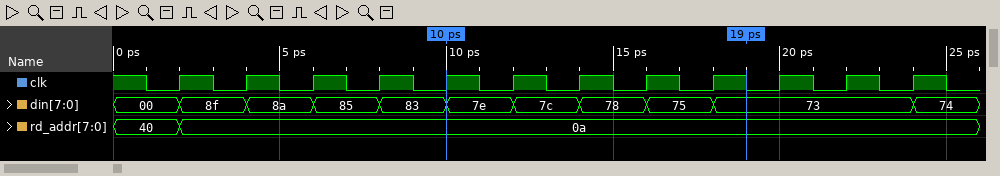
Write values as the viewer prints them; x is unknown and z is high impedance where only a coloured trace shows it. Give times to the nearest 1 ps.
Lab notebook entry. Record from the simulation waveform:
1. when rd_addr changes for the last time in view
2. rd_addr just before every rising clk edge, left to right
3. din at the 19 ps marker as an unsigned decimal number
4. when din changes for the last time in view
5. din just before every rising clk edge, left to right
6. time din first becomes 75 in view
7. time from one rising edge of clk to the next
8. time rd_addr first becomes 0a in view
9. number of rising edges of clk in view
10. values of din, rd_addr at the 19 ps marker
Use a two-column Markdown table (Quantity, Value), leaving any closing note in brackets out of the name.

| Quantity | Value |
|---|---|
| when rd_addr changes for the last time in view | 2 ps |
| rd_addr just before every rising clk edge, left to right | 40, 0a, 0a, 0a, 0a, 0a, 0a, 0a, 0a, 0a, 0a, 0a |
| din at the 19 ps marker as an unsigned decimal number | 115 |
| when din changes for the last time in view | 24 ps |
| din just before every rising clk edge, left to right | 00, 8f, 8a, 85, 83, 7e, 7c, 78, 75, 73, 73, 73 |
| time din first becomes 75 in view | 16 ps |
| time from one rising edge of clk to the next | 2 ps |
| time rd_addr first becomes 0a in view | 2 ps |
| number of rising edges of clk in view | 12 |
| values of din, rd_addr at the 19 ps marker | din=73, rd_addr=0a |
